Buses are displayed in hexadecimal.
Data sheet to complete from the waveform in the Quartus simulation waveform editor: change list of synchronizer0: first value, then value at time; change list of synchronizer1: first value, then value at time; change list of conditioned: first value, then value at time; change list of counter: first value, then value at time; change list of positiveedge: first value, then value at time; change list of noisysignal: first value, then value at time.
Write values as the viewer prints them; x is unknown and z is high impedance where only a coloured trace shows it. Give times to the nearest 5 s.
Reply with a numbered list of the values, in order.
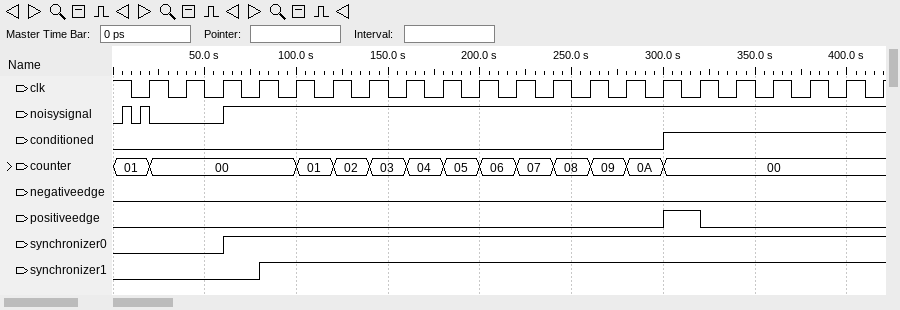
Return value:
1. 0, 1 at 60 s
2. 0, 1 at 80 s
3. 0, 1 at 300 s
4. 01, 00 at 20 s, 01 at 100 s, 02 at 120 s, 03 at 140 s, 04 at 160 s, 05 at 180 s, 06 at 200 s, 07 at 220 s, 08 at 240 s, 09 at 260 s, 0A at 280 s, 00 at 300 s
5. 0, 1 at 300 s, 0 at 320 s
6. 0, 1 at 5 s, 0 at 10 s, 1 at 15 s, 0 at 20 s, 1 at 60 s
